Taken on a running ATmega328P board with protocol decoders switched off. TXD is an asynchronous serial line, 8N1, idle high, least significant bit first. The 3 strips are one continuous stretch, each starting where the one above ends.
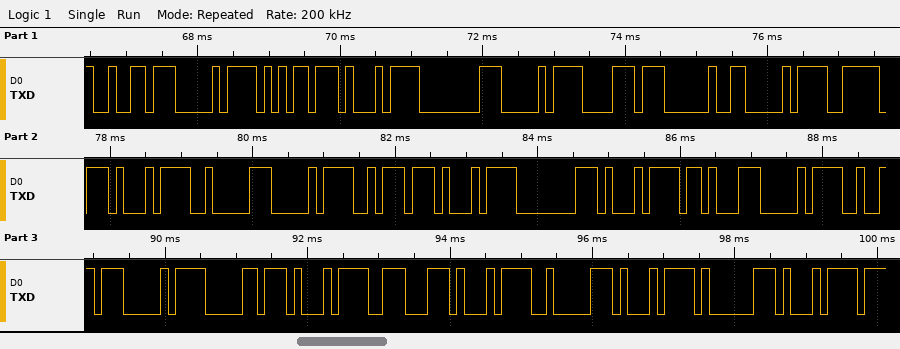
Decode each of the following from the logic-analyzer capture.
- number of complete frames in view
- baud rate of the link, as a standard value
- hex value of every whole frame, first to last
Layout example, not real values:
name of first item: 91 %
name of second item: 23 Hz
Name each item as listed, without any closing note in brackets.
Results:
number of complete frames in view: 29
baud rate of the link, as a standard value: 9600 baud
hex value of every whole frame, first to last: B2 D0 B5 D1 80 D0 B8 20 D0 BE D1 82 D0 BA D1 80 D1 8B D0 B2 D0 B0 D1 8E D1 82 D1 81 D1
